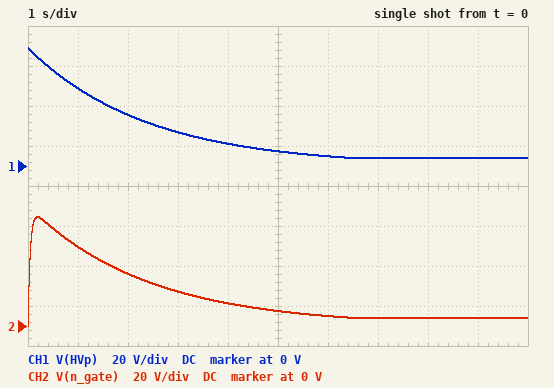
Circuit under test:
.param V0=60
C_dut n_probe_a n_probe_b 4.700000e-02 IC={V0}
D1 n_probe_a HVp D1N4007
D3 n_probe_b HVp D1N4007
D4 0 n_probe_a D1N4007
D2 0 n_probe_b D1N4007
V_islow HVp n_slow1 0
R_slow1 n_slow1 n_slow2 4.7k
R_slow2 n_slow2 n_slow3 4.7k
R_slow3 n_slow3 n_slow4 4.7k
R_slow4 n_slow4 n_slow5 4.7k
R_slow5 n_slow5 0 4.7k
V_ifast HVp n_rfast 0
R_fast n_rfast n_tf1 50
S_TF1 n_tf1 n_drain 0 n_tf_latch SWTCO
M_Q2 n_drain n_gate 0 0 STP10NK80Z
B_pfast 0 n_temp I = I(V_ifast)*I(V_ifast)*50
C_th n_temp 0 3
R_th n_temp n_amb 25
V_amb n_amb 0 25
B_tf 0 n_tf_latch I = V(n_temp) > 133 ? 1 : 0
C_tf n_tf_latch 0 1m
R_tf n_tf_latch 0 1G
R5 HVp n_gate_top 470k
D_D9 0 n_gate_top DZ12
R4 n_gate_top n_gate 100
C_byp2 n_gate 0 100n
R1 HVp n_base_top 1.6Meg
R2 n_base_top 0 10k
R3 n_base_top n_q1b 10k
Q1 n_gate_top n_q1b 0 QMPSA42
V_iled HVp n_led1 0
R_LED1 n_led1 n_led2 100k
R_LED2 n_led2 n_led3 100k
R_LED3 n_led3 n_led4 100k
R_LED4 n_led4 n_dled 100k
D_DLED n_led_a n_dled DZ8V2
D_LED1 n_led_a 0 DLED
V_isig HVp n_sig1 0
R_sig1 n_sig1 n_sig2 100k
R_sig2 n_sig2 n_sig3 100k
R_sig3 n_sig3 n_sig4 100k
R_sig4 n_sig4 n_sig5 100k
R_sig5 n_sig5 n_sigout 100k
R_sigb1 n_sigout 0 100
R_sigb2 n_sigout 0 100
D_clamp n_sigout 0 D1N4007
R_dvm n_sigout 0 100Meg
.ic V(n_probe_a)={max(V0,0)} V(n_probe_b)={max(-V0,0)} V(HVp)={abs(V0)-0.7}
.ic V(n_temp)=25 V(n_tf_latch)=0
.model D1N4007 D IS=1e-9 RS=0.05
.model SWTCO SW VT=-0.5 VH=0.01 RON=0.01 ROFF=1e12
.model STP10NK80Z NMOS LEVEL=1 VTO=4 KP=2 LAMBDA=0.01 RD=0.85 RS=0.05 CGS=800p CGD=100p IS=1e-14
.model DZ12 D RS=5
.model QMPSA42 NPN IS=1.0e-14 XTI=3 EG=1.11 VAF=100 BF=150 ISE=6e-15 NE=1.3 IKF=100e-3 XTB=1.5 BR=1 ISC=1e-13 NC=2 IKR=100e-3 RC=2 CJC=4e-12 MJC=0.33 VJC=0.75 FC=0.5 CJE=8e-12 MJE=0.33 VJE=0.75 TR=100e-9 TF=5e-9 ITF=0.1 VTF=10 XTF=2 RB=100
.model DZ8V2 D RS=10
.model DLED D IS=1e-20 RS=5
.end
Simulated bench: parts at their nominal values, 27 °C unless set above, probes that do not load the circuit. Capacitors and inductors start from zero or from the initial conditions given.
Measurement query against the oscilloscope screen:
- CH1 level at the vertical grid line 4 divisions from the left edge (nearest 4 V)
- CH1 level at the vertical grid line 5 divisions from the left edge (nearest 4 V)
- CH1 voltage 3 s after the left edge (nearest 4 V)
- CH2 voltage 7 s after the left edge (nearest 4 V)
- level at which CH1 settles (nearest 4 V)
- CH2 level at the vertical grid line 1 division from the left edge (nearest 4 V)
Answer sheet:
12 V
8 V
16 V
4 V
4 V
40 V
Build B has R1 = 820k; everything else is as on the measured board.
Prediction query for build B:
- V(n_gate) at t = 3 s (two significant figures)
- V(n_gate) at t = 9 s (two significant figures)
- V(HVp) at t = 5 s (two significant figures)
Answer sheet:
90 mV
91 mV
59 V
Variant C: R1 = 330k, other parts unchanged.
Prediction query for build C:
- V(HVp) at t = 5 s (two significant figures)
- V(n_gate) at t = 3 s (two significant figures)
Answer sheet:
59 V
38 mV
